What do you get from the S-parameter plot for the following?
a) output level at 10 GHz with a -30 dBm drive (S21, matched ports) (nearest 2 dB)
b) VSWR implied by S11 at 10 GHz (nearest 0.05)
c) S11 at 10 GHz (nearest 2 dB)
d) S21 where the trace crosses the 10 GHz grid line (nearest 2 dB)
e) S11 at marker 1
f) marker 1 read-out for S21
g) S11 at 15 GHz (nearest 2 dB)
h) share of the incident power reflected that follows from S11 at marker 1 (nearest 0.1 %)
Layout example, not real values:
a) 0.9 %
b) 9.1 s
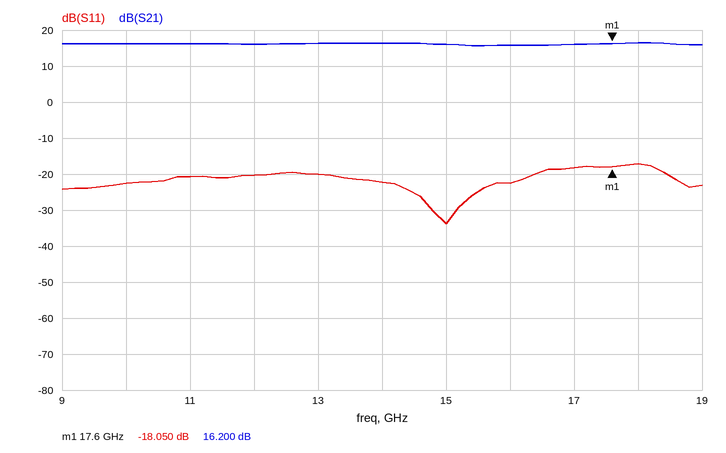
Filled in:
a) -14 dBm
b) 1.15
c) -22 dB
d) 16 dB
e) -18.050 dB
f) 16.200 dB
g) -34 dB
h) 1.6 %
